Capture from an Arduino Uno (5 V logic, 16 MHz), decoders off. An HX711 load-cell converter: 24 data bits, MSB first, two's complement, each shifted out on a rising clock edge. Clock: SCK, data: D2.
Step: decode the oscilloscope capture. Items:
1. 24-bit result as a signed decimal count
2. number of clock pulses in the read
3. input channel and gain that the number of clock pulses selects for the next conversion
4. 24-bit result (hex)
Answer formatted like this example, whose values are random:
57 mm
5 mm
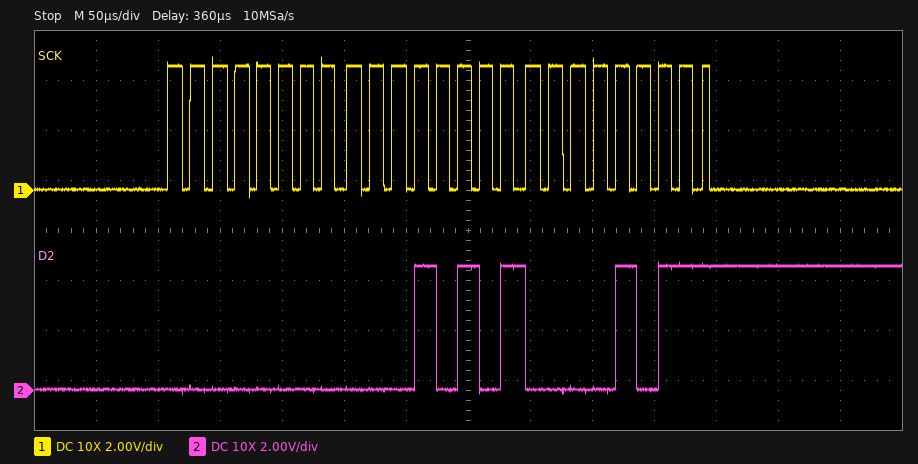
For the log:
5387
25
channel A, gain 128
0x00150B
